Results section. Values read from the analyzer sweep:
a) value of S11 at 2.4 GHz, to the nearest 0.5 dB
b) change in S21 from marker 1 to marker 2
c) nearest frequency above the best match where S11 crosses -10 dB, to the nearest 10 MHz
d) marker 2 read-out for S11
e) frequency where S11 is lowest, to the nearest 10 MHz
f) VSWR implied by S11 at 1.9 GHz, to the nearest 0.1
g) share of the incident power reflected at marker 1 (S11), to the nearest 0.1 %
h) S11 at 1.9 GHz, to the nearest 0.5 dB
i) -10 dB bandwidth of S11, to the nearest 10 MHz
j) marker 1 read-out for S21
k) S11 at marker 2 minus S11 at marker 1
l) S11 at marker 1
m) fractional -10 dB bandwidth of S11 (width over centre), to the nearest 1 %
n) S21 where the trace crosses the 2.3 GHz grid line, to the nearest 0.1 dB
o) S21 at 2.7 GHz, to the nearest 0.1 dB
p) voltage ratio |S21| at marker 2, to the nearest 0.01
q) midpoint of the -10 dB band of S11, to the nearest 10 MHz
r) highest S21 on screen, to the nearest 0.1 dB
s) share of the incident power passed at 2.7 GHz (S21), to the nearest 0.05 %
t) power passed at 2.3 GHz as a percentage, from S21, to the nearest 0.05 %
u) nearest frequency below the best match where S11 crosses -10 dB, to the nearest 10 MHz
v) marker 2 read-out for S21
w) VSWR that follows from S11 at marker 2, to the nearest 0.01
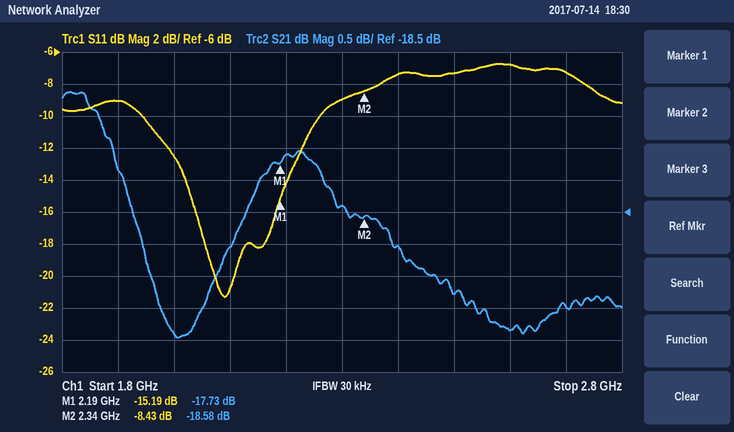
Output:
-7.5 dB
-0.85 dB
2.26 GHz
-8.43 dB
2.09 GHz
2.1
3.0 %
-9.0 dB
320 MHz
-17.73 dB
6.76 dB
-15.19 dB
15 %
-18.4 dB
-20.0 dB
0.12
2.10 GHz
-16.6 dB
1.00 %
1.45 %
1.94 GHz
-18.58 dB
2.22
